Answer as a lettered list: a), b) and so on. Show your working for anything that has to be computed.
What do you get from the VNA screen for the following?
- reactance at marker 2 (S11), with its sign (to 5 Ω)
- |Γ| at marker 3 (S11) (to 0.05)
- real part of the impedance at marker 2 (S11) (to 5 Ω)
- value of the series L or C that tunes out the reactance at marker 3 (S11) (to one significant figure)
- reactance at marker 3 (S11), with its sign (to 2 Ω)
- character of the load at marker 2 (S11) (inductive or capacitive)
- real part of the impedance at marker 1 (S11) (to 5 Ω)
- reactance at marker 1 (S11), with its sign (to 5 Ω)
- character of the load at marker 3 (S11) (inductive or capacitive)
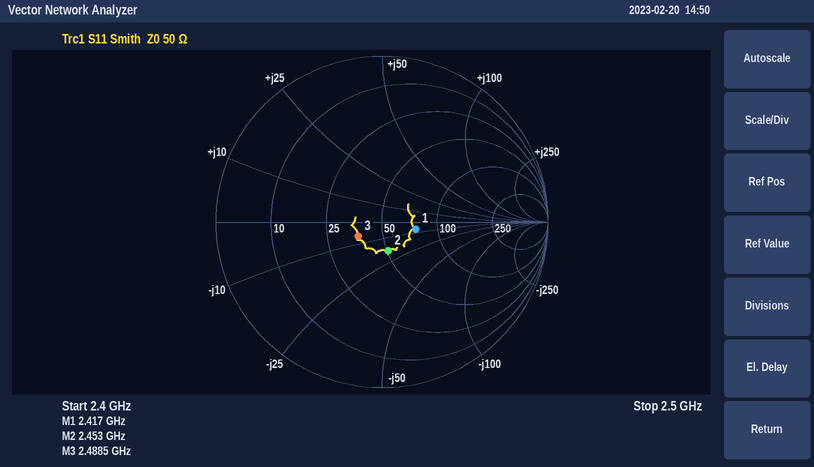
a) -20 Ω
b) 0.15
c) 50 Ω
d) L = 6 Ω/(2π × 2.4885 GHz) ≈ 384 pH, so 400 pH to one significant figure
e) -6 Ω
f) capacitive
g) 75 Ω
h) -5 Ω
i) capacitive
